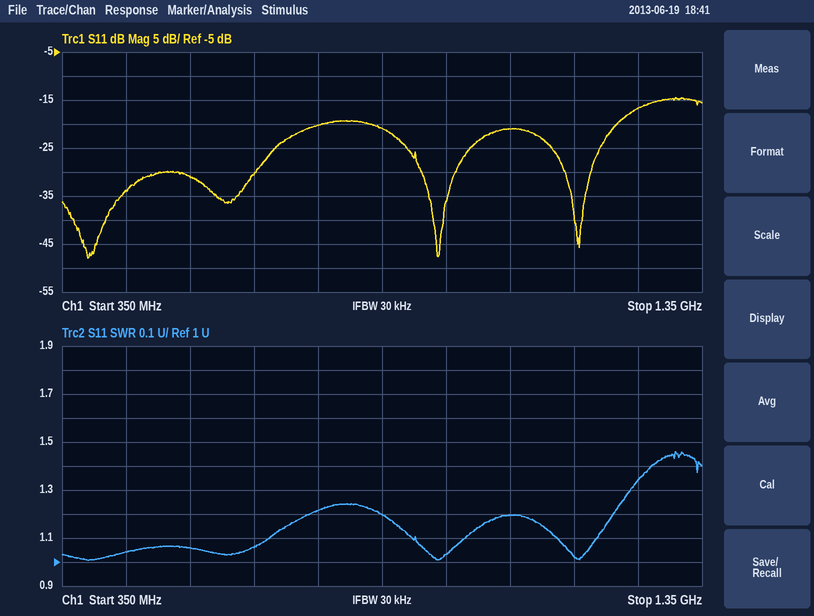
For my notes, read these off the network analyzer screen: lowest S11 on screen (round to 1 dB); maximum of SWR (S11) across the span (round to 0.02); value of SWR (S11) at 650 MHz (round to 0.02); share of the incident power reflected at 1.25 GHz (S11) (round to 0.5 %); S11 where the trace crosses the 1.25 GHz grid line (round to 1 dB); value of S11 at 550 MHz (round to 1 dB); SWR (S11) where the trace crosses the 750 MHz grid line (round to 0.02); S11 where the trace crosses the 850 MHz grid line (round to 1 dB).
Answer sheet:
-48 dB
1.46
1.06
2.0 %
-17 dB
-31 dB
1.22
-21 dB
